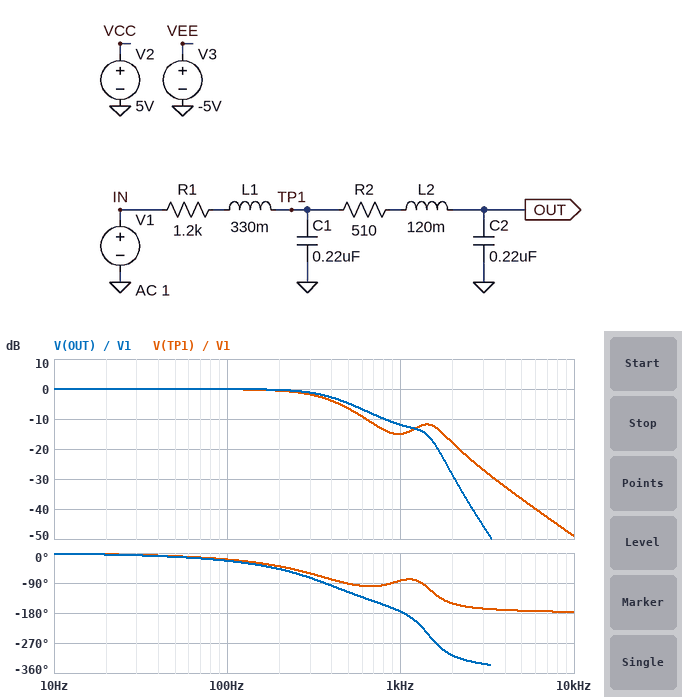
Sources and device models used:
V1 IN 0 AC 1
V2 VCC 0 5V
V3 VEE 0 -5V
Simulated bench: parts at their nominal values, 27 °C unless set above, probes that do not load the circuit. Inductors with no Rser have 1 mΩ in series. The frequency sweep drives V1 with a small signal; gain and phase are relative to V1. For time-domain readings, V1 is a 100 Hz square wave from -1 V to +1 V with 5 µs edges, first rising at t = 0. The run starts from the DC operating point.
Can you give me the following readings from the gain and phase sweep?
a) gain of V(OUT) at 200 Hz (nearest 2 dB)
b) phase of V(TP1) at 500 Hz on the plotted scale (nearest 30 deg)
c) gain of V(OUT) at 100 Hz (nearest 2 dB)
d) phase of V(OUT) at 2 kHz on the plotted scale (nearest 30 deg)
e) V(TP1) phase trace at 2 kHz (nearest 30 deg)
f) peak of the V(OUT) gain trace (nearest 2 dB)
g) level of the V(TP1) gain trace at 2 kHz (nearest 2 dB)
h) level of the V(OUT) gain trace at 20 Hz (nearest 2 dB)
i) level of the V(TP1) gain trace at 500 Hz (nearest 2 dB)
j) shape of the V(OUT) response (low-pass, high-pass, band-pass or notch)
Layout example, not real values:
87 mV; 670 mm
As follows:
0 dB; -90 deg; 0 dB; -300 deg; -150 deg; 0 dB; -18 dB; 0 dB; -6 dB; low-pass
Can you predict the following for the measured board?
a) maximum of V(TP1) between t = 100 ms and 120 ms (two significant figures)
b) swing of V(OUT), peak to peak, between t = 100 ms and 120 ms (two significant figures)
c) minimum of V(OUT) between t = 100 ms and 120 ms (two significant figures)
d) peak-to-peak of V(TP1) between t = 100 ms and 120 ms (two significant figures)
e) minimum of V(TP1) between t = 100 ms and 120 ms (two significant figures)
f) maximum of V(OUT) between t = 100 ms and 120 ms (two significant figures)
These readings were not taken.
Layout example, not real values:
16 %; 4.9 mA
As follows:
1.1 V; 2.1 V; -1.1 V; 2.1 V; -1.1 V; 1.1 V
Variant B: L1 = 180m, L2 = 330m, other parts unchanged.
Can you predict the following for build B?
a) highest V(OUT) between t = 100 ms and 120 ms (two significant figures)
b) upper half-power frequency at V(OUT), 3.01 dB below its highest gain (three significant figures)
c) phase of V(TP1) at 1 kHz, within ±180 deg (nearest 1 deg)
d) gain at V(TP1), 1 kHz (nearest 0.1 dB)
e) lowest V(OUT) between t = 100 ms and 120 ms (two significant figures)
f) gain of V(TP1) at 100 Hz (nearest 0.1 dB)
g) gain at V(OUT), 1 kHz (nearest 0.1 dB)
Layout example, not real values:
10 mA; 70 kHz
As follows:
1.0 V; 525 Hz; -68 deg; -1.9 dB; -1.0 V; -0.3 dB; -7.9 dB
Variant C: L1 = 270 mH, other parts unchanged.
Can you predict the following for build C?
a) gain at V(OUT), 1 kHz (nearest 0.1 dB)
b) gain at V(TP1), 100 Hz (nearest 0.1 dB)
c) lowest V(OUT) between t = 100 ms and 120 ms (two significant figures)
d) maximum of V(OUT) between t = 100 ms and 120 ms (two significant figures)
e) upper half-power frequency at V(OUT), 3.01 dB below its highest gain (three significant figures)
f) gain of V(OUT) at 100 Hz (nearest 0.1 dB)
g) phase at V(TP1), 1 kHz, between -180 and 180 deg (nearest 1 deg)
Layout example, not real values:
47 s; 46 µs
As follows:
-10.9 dB; -0.2 dB; -1.0 V; 1.0 V; 408 Hz; -0.1 dB; -76 deg
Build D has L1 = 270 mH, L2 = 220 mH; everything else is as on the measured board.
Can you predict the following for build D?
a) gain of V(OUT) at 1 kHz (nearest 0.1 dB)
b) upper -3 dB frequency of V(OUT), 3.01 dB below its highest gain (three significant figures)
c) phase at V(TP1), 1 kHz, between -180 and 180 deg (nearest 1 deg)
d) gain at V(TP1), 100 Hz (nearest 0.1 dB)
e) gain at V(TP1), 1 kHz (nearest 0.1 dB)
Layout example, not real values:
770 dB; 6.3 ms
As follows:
-7.7 dB; 446 Hz; -57 deg; -0.2 dB; -6.5 dB
